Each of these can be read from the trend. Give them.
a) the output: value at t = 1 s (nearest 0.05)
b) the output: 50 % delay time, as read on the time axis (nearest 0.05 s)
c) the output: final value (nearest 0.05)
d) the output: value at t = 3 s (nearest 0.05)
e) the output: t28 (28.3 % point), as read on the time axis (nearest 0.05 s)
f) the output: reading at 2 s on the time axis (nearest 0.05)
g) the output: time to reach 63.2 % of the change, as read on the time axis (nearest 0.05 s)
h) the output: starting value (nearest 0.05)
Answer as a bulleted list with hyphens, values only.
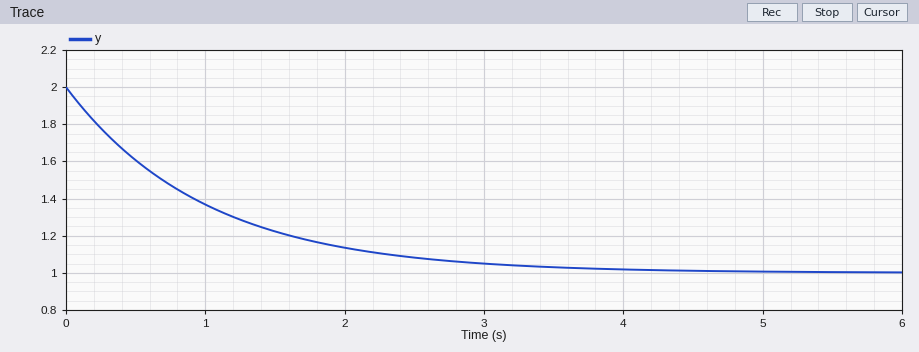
- 1.35
- 0.70 s
- 1.00
- 1.05
- 0.35 s
- 1.15
- 1.00 s
- 2.00
